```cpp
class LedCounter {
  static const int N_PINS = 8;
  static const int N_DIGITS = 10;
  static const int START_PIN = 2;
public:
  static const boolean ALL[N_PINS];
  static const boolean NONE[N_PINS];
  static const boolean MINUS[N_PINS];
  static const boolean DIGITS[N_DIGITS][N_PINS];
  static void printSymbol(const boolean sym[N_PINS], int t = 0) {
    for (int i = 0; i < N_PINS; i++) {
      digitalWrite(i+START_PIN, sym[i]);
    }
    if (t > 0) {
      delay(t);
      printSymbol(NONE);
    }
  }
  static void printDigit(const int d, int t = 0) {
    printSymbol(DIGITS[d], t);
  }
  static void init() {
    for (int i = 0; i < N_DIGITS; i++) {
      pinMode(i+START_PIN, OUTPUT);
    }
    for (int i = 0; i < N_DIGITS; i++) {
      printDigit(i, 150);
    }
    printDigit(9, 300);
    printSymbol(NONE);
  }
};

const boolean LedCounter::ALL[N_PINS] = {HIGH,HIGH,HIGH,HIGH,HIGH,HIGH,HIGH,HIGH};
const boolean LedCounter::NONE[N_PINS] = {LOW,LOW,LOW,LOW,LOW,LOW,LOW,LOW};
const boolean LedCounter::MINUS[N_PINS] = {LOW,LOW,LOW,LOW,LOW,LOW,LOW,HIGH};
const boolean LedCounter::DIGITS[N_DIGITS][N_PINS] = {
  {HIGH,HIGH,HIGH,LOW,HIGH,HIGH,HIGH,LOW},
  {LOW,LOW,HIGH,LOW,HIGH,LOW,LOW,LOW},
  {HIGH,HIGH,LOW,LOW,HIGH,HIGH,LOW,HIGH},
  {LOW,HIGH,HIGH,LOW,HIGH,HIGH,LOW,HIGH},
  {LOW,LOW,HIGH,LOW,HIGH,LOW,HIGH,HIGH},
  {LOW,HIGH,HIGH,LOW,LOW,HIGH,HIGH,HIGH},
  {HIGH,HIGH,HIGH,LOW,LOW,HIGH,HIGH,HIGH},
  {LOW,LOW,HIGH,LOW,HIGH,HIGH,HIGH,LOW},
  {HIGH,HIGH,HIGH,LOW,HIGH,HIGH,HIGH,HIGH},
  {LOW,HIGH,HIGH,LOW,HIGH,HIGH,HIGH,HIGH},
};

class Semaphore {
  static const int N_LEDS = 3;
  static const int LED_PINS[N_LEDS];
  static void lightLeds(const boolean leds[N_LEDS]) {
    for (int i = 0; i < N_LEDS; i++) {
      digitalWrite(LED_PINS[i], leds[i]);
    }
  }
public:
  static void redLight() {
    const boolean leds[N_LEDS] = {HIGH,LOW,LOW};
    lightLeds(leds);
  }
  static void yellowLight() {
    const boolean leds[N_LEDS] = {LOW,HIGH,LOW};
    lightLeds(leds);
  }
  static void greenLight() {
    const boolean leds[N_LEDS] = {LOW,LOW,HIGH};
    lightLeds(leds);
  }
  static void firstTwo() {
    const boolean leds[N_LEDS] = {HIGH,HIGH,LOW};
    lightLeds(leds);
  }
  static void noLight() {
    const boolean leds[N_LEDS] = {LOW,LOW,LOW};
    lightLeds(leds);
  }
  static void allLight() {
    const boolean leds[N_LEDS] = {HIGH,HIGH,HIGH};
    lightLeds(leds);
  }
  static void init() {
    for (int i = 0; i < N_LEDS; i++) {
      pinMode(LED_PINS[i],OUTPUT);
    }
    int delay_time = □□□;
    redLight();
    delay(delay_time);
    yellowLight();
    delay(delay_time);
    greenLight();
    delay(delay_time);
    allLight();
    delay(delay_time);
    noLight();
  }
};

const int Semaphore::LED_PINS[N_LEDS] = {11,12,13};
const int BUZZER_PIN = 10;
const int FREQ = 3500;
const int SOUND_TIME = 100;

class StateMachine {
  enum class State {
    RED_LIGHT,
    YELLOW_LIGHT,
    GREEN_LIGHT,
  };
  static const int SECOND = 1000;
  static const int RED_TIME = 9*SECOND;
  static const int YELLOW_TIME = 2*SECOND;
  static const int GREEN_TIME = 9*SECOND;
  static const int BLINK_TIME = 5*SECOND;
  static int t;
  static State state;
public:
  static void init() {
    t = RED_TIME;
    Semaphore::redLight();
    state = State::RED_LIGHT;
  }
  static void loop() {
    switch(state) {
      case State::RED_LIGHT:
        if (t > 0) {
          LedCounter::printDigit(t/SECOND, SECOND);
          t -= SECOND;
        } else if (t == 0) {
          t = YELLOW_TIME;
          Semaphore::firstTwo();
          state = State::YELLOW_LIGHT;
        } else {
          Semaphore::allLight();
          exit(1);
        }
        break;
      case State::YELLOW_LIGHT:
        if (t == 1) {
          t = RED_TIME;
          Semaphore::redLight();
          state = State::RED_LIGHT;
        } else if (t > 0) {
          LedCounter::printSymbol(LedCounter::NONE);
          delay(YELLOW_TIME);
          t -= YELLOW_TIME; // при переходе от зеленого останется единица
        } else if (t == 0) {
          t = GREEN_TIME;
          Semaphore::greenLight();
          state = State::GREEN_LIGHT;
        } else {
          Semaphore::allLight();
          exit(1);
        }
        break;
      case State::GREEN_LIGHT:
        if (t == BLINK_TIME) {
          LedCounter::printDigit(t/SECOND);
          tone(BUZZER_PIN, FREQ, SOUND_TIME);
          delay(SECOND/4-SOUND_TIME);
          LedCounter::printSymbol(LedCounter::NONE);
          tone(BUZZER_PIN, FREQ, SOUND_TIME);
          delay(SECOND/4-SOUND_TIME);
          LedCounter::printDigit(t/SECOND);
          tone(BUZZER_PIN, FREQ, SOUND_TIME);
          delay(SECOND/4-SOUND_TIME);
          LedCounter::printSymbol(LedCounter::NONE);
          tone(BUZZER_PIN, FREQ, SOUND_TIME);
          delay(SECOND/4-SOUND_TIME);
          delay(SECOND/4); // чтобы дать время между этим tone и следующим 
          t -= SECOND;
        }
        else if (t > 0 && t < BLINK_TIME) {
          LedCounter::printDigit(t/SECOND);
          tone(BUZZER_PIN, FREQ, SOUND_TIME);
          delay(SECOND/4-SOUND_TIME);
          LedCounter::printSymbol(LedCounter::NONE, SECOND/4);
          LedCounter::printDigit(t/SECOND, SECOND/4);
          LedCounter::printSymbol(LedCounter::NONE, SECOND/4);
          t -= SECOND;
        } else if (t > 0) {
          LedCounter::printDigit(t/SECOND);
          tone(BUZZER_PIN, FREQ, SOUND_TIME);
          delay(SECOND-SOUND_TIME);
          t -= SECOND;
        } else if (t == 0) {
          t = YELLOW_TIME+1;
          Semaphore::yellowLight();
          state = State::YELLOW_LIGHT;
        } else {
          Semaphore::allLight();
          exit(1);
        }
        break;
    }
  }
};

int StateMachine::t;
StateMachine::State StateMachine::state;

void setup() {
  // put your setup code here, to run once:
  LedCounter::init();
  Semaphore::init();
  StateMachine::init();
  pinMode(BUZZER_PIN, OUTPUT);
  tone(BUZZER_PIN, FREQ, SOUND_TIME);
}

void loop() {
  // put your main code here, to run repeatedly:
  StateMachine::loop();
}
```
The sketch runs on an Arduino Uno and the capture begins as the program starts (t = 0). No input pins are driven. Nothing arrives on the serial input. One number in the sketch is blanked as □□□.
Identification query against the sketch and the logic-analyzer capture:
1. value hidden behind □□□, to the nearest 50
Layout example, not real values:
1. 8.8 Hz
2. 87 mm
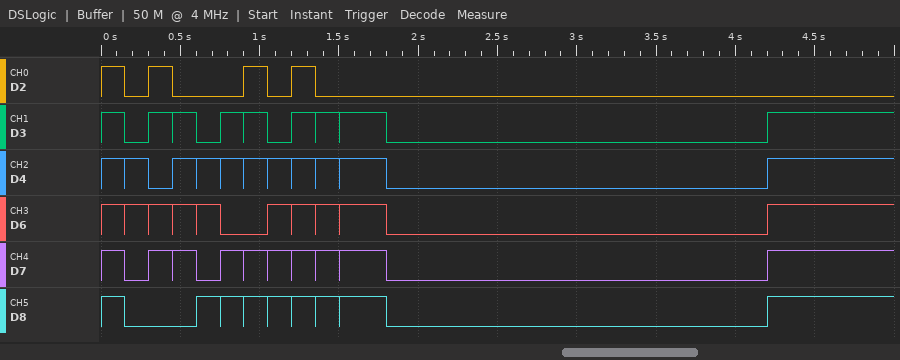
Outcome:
1. 600
